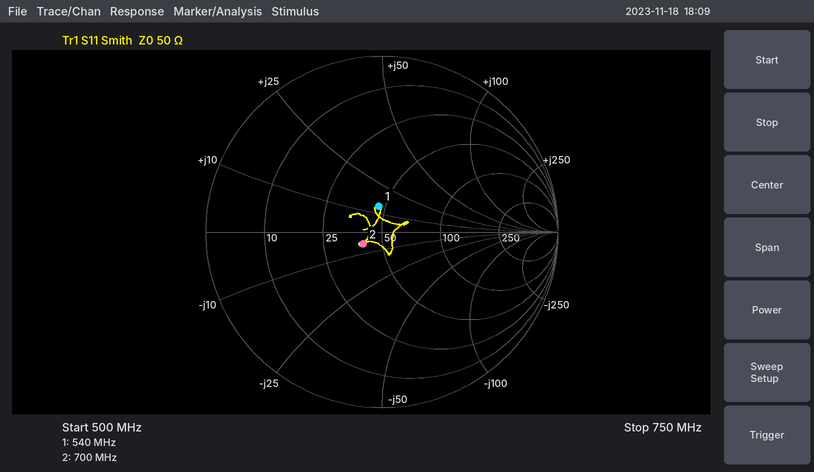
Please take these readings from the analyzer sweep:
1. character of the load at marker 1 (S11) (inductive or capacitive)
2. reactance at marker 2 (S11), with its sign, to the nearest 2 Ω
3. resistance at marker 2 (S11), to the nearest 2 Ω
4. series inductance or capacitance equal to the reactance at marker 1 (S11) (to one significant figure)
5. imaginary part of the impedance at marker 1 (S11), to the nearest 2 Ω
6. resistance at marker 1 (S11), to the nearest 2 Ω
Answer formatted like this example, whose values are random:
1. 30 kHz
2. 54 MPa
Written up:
1. inductive
2. -6 Ω
3. 40 Ω
4. 4 nH
5. +14 Ω
6. 46 Ω
